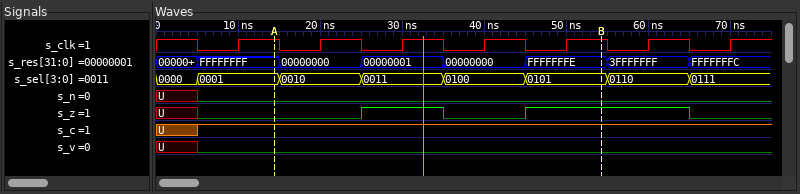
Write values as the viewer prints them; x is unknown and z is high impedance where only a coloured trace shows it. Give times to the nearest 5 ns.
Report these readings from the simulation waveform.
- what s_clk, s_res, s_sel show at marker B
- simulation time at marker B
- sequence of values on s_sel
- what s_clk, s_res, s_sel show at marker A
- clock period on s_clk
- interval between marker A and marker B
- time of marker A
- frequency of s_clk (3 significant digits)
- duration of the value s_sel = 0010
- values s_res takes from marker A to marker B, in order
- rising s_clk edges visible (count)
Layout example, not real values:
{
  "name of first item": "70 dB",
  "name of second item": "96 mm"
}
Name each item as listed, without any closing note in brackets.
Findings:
{
  "what s_clk, s_res, s_sel show at marker B": "s_clk=1, s_res=FFFFFFFE, s_sel=0101",
  "simulation time at marker B": "55 ns",
  "sequence of values on s_sel": "0000, 0001, 0010, 0011, 0100, 0101, 0110, 0111",
  "what s_clk, s_res, s_sel show at marker A": "s_clk=1, s_res=FFFFFFFF, s_sel=0001",
  "clock period on s_clk": "10 ns",
  "interval between marker A and marker B": "40 ns",
  "time of marker A": "15 ns",
  "frequency of s_clk": "100 MHz",
  "duration of the value s_sel = 0010": "10 ns",
  "values s_res takes from marker A to marker B, in order": "FFFFFFFF, 00000000, 00000001, 00000000, FFFFFFFE",
  "rising s_clk edges visible": "7"
}
